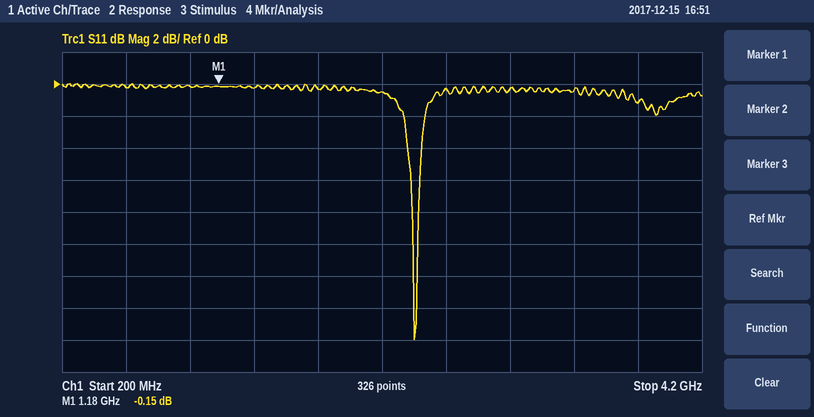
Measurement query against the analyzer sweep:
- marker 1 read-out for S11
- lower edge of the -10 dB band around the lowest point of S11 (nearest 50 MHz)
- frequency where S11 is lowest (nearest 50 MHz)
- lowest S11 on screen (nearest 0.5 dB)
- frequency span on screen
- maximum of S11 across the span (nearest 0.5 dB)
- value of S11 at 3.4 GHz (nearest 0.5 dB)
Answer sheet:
-0.15 dB
2.40 GHz
2.40 GHz
-16.0 dB
4 GHz
0.0 dB
-0.5 dB
